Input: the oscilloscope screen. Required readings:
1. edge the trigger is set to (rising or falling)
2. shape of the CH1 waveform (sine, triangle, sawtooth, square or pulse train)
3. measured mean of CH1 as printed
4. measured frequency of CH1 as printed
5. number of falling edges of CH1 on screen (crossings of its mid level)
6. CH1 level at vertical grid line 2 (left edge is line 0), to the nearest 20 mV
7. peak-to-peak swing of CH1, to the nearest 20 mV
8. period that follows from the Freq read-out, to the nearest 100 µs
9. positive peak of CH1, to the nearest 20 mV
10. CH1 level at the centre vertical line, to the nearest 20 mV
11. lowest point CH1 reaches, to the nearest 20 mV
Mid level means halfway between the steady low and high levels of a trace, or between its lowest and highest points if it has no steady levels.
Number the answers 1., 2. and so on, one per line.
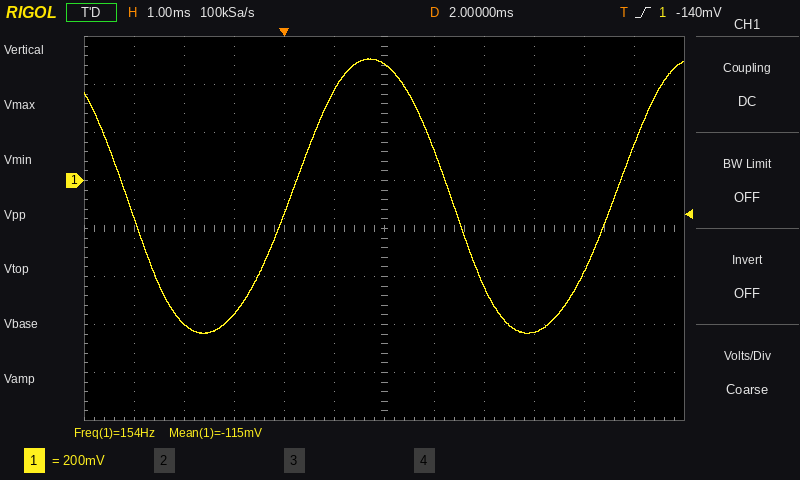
1. rising
2. sine
3. -115 mV
4. 154 Hz
5. 2
6. -600 mV
7. 1.14 V
8. 6.5 ms
9. 500 mV
10. 480 mV
11. -640 mV
